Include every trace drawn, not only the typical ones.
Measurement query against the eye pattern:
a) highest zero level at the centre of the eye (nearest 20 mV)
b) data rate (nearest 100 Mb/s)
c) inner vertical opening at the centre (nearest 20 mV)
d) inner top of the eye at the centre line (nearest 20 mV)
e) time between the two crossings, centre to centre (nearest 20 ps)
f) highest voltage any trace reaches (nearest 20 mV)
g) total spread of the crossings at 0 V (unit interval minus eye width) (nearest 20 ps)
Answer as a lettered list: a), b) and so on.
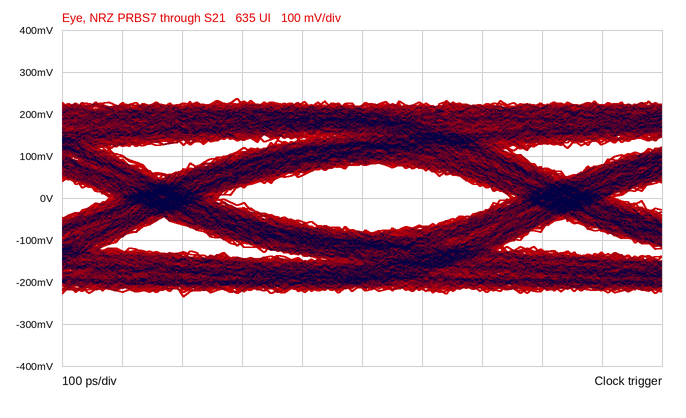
a) -80 mV
b) 1.5 Gb/s
c) 160 mV
d) 80 mV
e) 660 ps
f) 240 mV
g) 180 ps
